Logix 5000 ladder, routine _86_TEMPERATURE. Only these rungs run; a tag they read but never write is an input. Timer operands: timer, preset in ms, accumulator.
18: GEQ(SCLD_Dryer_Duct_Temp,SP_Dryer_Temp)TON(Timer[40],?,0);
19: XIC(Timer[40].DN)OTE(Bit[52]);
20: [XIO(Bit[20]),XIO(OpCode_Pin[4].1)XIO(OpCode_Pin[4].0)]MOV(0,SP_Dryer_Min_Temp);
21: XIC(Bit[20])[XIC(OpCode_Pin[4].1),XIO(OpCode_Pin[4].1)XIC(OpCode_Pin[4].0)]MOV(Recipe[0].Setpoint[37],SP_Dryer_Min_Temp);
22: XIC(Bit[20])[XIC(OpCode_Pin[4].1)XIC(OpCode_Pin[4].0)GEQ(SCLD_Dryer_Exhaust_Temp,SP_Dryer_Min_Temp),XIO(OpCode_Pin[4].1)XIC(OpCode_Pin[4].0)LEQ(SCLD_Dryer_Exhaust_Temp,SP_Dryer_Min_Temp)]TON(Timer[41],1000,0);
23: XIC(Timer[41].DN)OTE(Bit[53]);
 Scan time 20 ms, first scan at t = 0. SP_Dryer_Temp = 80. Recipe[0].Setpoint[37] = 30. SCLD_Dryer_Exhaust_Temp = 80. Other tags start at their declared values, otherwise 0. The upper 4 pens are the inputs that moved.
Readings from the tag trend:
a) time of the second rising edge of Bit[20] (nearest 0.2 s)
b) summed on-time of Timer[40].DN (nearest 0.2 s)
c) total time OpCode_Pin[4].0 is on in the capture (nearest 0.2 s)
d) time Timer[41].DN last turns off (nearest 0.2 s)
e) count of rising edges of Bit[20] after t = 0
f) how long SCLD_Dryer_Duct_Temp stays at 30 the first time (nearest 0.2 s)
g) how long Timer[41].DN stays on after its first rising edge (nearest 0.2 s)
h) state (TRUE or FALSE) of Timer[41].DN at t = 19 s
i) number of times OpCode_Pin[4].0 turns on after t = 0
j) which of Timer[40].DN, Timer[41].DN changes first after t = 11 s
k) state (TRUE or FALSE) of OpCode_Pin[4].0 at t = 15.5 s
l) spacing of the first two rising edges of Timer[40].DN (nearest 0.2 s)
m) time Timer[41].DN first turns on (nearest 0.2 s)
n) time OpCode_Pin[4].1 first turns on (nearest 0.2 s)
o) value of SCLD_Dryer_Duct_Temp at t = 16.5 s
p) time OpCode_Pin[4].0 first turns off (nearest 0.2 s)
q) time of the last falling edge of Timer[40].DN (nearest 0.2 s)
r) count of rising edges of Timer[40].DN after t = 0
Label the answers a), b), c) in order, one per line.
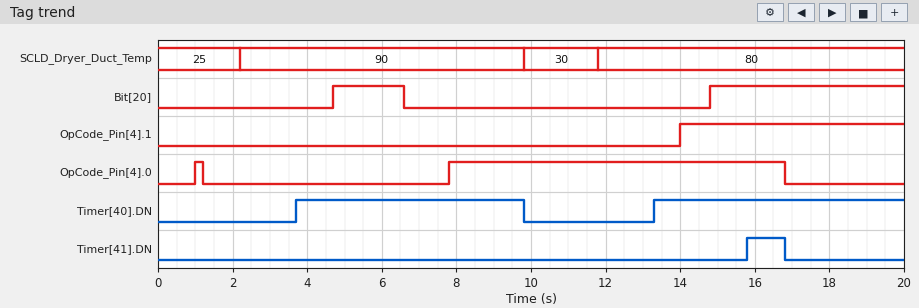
a) 14.8 s
b) 12.8 s
c) 9.2 s
d) 16.8 s
e) 2
f) 2.0 s
g) 1.0 s
h) FALSE
i) 2
j) Timer[40].DN
k) TRUE
l) 9.6 s
m) 15.8 s
n) 14.0 s
o) 80
p) 1.2 s
q) 9.8 s
r) 2
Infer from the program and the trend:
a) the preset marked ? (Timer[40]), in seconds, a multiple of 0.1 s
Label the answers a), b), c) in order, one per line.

a) 1.5 s
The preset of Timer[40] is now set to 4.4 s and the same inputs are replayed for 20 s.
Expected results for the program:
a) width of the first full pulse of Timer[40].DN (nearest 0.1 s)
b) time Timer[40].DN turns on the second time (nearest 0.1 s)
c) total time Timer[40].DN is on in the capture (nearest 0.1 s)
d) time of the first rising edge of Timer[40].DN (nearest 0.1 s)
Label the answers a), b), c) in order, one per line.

a) 3.2 s
b) 16.2 s
c) 7.0 s
d) 6.6 s
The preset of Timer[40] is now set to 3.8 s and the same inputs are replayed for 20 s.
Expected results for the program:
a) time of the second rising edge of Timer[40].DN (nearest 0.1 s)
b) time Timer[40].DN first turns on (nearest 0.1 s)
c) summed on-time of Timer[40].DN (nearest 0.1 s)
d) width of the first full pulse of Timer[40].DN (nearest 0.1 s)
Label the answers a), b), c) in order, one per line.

a) 15.6 s
b) 6.0 s
c) 8.2 s
d) 3.8 s
